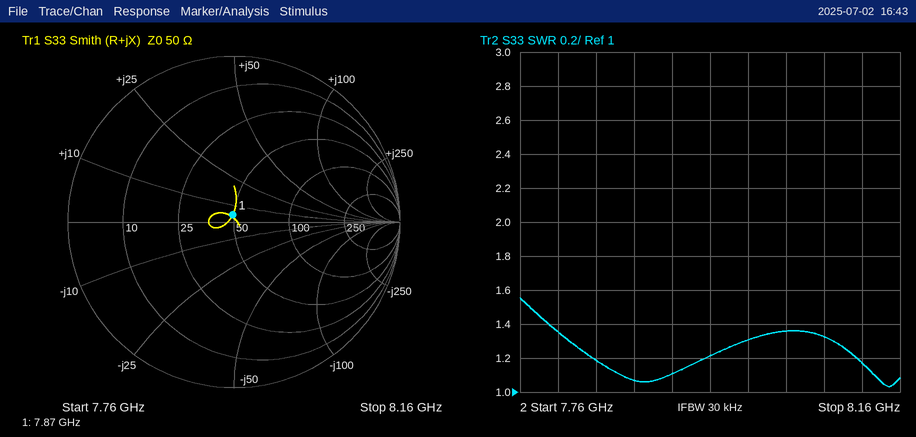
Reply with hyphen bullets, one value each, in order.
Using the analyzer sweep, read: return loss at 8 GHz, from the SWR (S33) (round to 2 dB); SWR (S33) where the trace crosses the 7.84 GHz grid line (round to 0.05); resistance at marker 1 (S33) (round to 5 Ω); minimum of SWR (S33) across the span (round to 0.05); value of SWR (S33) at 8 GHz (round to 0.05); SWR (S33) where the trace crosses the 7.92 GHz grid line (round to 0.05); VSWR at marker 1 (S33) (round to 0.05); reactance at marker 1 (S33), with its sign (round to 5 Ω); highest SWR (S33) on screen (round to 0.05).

- 18 dB
- 1.20
- 50 Ω
- 1.05
- 1.30
- 1.10
- 1.10
- +5 Ω
- 1.55
